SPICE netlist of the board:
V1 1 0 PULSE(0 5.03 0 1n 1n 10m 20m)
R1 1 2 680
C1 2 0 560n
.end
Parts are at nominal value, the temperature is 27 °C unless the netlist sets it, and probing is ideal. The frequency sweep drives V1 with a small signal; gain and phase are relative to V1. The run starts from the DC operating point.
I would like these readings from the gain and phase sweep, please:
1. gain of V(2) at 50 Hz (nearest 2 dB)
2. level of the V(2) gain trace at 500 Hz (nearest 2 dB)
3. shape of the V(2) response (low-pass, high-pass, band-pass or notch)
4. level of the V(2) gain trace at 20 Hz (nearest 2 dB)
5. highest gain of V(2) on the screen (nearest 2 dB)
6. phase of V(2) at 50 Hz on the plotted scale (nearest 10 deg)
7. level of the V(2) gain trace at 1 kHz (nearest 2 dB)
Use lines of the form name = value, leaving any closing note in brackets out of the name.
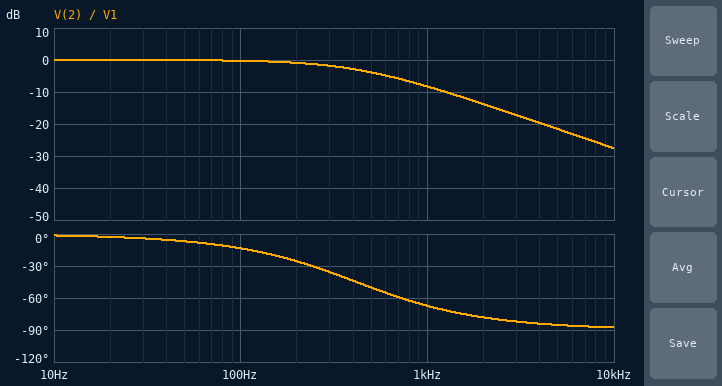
gain of V(2) at 50 Hz = 0 dB
level of the V(2) gain trace at 500 Hz = -4 dB
shape of the V(2) response = low-pass
level of the V(2) gain trace at 20 Hz = 0 dB
highest gain of V(2) on the screen = 0 dB
phase of V(2) at 50 Hz on the plotted scale = -10 deg
level of the V(2) gain trace at 1 kHz = -8 dB
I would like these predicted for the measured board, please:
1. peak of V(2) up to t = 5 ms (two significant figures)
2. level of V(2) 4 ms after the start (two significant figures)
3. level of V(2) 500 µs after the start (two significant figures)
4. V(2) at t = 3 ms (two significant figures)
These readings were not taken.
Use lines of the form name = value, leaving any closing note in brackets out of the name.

peak of V(2) up to t = 5 ms = 5.0 V
level of V(2) 4 ms after the start = 5.0 V
level of V(2) 500 µs after the start = 3.7 V
V(2) at t = 3 ms = 5.0 V
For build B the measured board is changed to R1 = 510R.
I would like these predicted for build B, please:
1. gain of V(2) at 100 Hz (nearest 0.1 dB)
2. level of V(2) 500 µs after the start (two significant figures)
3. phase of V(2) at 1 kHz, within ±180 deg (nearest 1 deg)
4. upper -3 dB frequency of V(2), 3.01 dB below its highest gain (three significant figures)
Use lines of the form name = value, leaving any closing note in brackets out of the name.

gain of V(2) at 100 Hz = -0.1 dB
level of V(2) 500 µs after the start = 4.2 V
phase of V(2) at 1 kHz, within ±180 deg = -61 deg
upper -3 dB frequency of V(2), 3.01 dB below its highest gain = 557 Hz
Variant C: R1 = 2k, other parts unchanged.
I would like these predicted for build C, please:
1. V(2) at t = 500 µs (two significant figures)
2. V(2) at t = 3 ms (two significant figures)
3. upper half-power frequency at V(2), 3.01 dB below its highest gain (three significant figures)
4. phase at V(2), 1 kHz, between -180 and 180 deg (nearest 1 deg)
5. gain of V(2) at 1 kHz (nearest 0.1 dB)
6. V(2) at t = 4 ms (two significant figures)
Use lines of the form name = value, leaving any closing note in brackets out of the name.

V(2) at t = 500 µs = 1.8 V
V(2) at t = 3 ms = 4.7 V
upper half-power frequency at V(2), 3.01 dB below its highest gain = 142 Hz
phase at V(2), 1 kHz, between -180 and 180 deg = -82 deg
gain of V(2) at 1 kHz = -17.0 dB
V(2) at t = 4 ms = 4.9 V
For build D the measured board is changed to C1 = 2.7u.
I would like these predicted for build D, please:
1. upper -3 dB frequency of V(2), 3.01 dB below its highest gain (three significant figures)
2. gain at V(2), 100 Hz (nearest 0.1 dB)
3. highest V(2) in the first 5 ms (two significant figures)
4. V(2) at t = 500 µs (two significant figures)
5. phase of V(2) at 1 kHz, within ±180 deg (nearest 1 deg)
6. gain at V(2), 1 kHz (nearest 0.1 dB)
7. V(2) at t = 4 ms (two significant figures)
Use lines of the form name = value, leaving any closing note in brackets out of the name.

upper -3 dB frequency of V(2), 3.01 dB below its highest gain = 86.7 Hz
gain at V(2), 100 Hz = -3.7 dB
highest V(2) in the first 5 ms = 4.7 V
V(2) at t = 500 µs = 1.2 V
phase of V(2) at 1 kHz, within ±180 deg = -85 deg
gain at V(2), 1 kHz = -21.3 dB
V(2) at t = 4 ms = 4.5 V
